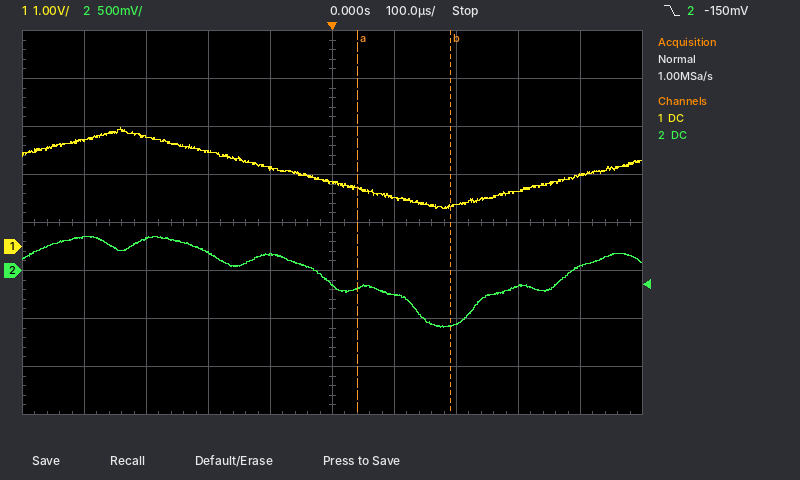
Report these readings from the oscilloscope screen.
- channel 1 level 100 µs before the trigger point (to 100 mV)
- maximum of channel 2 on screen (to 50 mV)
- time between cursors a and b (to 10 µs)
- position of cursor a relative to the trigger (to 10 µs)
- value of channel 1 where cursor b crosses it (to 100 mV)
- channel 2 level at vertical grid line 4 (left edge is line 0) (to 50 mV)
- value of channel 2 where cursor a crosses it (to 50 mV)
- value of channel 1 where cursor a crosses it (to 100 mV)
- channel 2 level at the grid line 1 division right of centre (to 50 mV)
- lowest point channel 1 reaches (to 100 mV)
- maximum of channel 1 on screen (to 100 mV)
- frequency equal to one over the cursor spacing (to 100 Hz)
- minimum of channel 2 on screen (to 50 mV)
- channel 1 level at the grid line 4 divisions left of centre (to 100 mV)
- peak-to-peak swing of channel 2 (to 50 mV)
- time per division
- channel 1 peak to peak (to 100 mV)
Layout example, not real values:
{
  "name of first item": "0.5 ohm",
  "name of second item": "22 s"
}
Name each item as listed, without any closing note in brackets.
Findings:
{
  "channel 1 level 100 µs before the trigger point": "1.6 V",
  "maximum of channel 2 on screen": "350 mV",
  "time between cursors a and b": "150 µs",
  "position of cursor a relative to the trigger": "+40 µs",
  "value of channel 1 where cursor b crosses it": "800 mV",
  "channel 2 level at vertical grid line 4 (left edge is line 0)": "150 mV",
  "value of channel 2 where cursor a crosses it": "-200 mV",
  "value of channel 1 where cursor a crosses it": "1.2 V",
  "channel 2 level at the grid line 1 division right of centre": "-250 mV",
  "lowest point channel 1 reaches": "800 mV",
  "maximum of channel 1 on screen": "2.5 V",
  "frequency equal to one over the cursor spacing": "6.7 kHz",
  "minimum of channel 2 on screen": "-600 mV",
  "channel 1 level at the grid line 4 divisions left of centre": "2.2 V",
  "peak-to-peak swing of channel 2": "950 mV",
  "time per division": "100 µs",
  "channel 1 peak to peak": "1.7 V"
}
